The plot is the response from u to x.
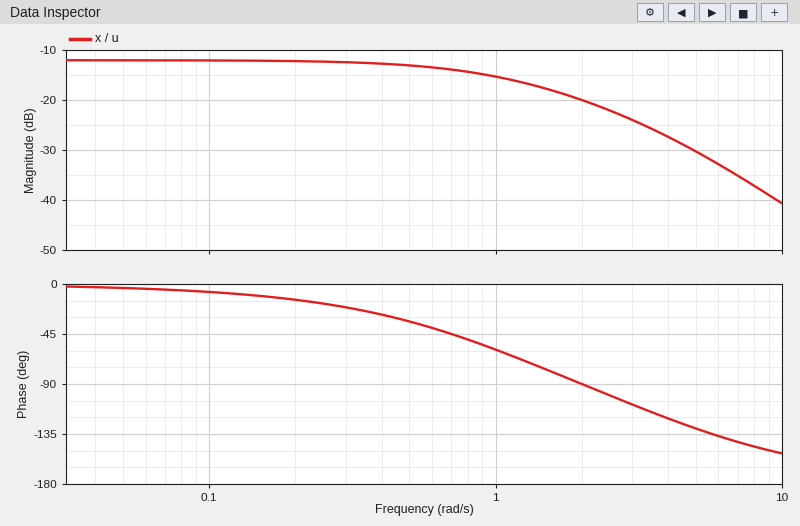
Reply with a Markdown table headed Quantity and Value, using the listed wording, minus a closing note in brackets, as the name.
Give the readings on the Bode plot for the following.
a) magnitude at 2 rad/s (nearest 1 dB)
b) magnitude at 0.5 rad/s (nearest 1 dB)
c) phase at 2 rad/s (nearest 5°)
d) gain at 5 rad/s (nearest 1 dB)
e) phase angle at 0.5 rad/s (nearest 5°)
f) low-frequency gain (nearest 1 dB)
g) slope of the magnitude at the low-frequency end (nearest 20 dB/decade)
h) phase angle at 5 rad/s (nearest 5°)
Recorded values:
| Quantity | Value |
|---|---|
| magnitude at 2 rad/s | -20 dB |
| magnitude at 0.5 rad/s | -13 dB |
| phase at 2 rad/s | -90° |
| gain at 5 rad/s | -30 dB |
| phase angle at 0.5 rad/s | -35° |
| low-frequency gain | -12 dB |
| slope of the magnitude at the low-frequency end | 0 dB/decade |
| phase angle at 5 rad/s | -130° |
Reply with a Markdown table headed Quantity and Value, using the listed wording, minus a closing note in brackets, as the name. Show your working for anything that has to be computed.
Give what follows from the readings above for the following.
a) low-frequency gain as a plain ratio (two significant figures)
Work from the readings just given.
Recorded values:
| Quantity | Value |
|---|---|
| low-frequency gain as a plain ratio | 10^(-12 / 20) = 0.25 |
